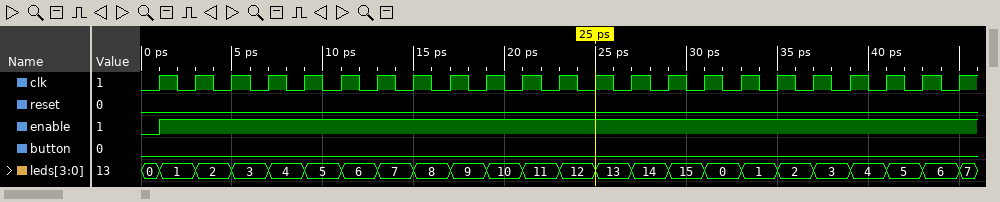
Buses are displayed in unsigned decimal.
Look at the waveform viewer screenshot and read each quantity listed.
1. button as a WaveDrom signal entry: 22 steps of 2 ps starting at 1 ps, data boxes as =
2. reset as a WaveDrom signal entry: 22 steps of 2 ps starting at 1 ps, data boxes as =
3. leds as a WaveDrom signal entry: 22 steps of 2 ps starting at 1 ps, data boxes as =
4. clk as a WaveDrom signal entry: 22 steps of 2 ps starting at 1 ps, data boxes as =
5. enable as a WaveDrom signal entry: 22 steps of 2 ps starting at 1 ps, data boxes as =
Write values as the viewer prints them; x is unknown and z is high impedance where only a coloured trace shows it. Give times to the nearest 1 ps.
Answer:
{name: 'button', wave: '0.....................'}
{name: 'reset', wave: '0.....................'}
{name: 'leds', wave: '======================', data: '1 2 3 4 5 6 7 8 9 10 11 12 13 14 15 0 1 2 3 4 5 6'}
{name: 'clk', wave: 'p.....................'}
{name: 'enable', wave: '1.....................'}
